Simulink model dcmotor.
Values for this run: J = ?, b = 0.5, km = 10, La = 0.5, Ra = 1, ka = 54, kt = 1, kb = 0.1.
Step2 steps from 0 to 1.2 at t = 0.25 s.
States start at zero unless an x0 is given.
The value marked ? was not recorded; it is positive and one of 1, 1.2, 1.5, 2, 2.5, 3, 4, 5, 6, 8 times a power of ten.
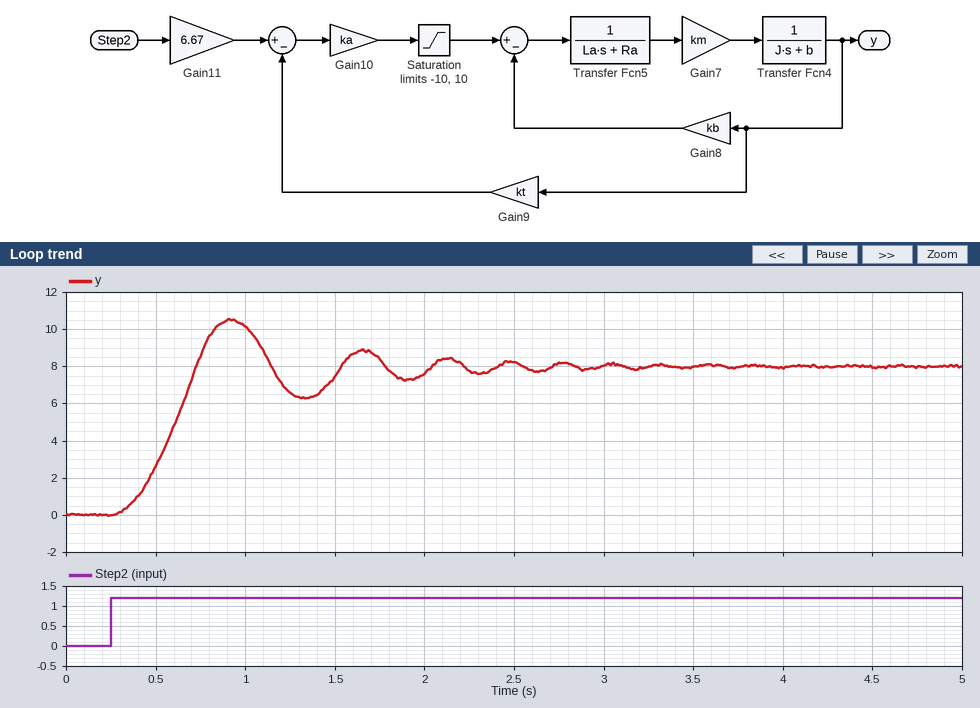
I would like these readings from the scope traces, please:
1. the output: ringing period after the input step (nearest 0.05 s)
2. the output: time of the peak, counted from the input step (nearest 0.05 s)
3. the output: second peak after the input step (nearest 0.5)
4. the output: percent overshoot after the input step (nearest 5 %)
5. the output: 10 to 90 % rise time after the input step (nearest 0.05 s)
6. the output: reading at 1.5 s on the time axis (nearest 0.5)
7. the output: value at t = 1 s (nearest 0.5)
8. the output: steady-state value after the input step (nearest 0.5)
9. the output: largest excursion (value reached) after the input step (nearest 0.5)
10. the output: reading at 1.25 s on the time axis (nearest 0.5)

0.75 s
0.65 s
9.0
30 %
0.30 s
7.5
10.0
8.0
10.5
6.5
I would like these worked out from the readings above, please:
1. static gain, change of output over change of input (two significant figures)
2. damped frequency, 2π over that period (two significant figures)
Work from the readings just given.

6.7
8.4 rad/s
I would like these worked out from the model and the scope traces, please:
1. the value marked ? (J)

2
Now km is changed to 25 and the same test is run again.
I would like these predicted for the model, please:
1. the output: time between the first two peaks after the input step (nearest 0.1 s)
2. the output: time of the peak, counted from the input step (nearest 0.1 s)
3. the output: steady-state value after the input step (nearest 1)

0.6 s
0.4 s
8
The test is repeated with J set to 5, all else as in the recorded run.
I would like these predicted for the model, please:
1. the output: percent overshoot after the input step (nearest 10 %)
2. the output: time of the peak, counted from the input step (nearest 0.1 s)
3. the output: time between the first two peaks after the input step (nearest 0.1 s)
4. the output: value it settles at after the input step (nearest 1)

20 %
1.1 s
0.9 s
8
